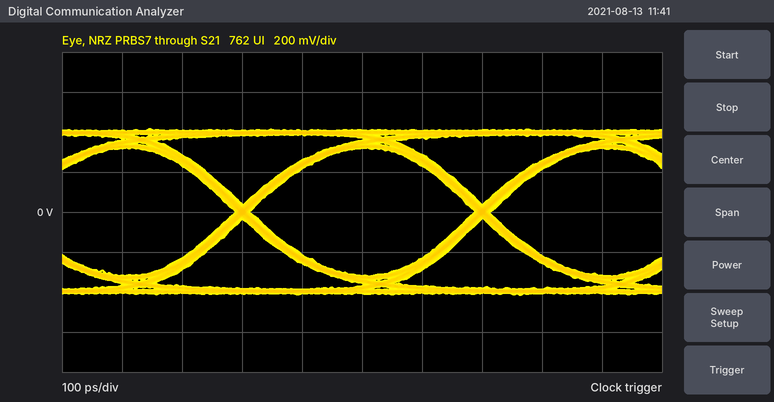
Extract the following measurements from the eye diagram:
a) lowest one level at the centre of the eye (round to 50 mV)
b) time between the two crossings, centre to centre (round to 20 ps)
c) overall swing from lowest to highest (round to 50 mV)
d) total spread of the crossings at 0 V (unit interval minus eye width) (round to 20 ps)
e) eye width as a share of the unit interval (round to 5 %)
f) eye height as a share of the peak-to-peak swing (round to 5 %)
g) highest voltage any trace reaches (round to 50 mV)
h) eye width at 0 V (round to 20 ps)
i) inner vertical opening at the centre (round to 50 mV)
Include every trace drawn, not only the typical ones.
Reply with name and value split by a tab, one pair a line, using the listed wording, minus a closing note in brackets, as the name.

lowest one level at the centre of the eye	300 mV
time between the two crossings, centre to centre	400 ps
overall swing from lowest to highest	850 mV
total spread of the crossings at 0 V (unit interval minus eye width)	20 ps
eye width as a share of the unit interval	95 %
eye height as a share of the peak-to-peak swing	75 %
highest voltage any trace reaches	400 mV
eye width at 0 V	380 ps
inner vertical opening at the centre	650 mV
